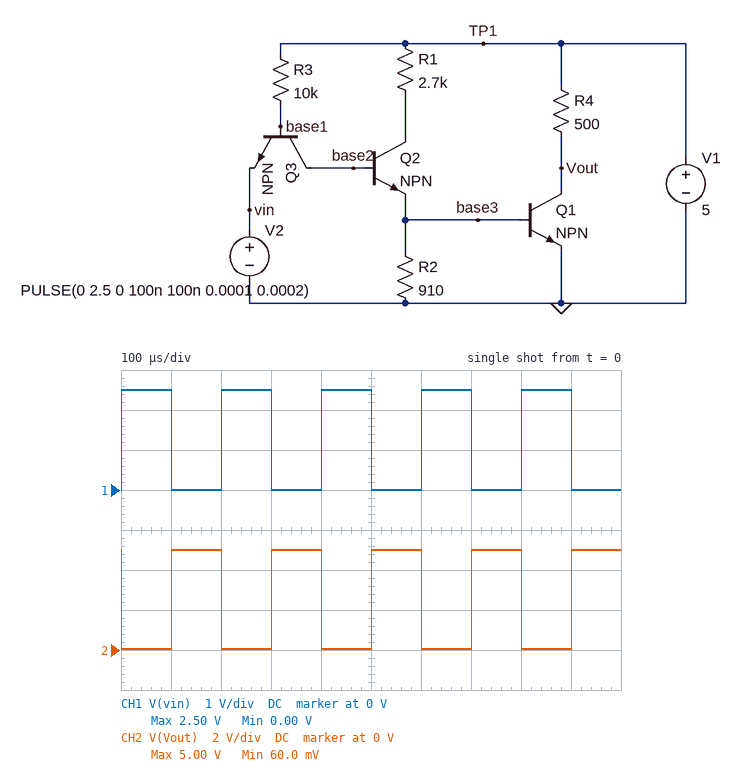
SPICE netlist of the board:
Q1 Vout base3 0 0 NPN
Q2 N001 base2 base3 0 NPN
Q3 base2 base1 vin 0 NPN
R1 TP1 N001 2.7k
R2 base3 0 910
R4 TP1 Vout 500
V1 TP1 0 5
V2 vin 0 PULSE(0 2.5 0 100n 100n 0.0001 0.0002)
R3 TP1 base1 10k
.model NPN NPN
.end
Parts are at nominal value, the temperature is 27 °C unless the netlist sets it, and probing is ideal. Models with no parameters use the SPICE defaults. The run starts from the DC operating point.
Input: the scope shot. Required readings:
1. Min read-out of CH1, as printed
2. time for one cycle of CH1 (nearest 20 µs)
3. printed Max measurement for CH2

0.00 V
200 µs
5.00 V
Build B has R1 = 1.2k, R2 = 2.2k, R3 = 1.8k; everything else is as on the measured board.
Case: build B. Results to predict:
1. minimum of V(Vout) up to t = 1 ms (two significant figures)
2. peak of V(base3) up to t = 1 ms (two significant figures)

34 mV
850 mV
